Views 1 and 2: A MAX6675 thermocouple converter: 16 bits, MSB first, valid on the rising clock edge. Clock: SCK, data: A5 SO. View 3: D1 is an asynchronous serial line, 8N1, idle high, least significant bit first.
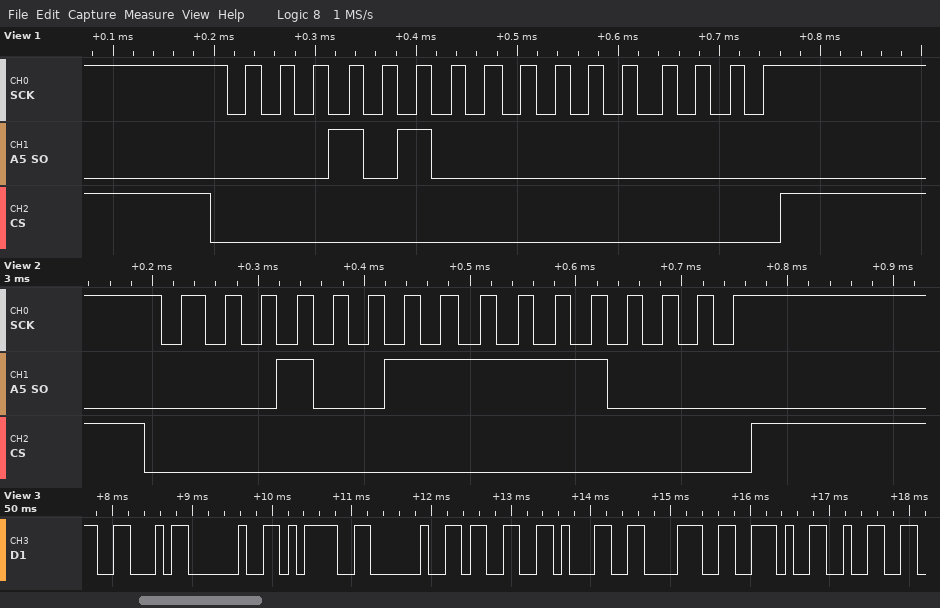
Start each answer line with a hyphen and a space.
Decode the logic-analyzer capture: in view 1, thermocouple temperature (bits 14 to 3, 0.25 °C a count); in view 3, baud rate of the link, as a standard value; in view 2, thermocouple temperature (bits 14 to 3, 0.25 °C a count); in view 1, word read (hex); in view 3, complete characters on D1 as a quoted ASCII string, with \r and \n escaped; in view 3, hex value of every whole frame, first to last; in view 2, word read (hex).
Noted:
- 160.00 °C
- 9600 baud
- 159.50 °C
- 0x1400
- "F = 318.2"
- 46 20 3D 20 33 31 38 2E 32
- 0x13F0
